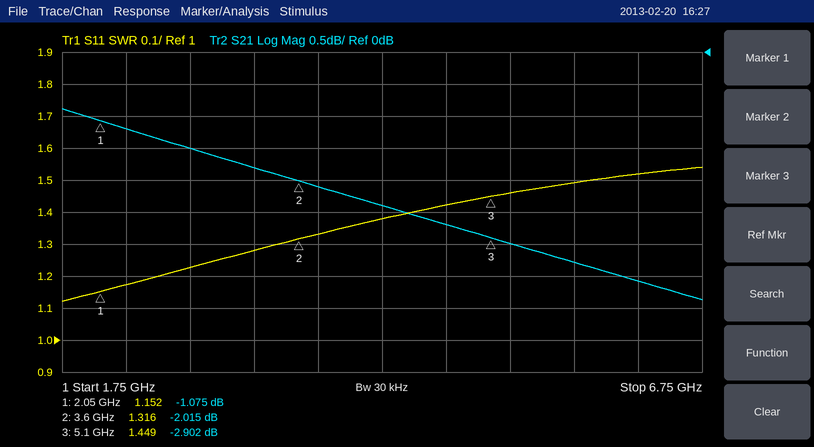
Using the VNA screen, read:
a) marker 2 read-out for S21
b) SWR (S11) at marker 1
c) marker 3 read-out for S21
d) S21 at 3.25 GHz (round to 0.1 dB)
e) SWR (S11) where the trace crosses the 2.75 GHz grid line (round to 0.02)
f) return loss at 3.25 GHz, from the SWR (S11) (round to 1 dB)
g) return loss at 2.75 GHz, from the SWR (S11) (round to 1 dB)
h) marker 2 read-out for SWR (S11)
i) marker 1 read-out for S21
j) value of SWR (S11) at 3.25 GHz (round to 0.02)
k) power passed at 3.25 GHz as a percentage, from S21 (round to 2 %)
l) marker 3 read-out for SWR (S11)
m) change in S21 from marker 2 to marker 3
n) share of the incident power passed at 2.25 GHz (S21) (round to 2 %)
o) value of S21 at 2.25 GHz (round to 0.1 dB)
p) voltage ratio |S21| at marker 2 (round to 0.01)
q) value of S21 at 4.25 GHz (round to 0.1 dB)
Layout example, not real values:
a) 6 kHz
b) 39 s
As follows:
a) -2.015 dB
b) 1.152
c) -2.902 dB
d) -1.8 dB
e) 1.22
f) 18 dB
g) 20 dB
h) 1.316
i) -1.075 dB
j) 1.28
k) 66 %
l) 1.449
m) -0.887 dB
n) 76 %
o) -1.2 dB
p) 0.79
q) -2.4 dB
